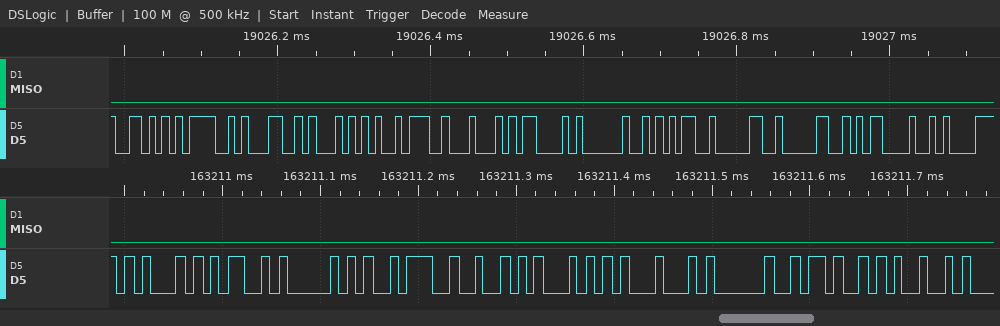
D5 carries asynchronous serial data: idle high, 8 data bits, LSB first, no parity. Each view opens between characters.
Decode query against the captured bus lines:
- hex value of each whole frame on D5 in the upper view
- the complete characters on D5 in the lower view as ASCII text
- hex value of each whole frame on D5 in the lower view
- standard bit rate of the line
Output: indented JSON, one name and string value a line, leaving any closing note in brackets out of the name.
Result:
{
  "hex value of each whole frame on D5 in the upper view": "56, 4F, 4C, 54, 3A, 44, 43, 20, 35, 30, 30, 0D, 0A",
  "the complete characters on D5 in the lower view as ASCII text": "\"EMP:RTD KI\"",
  "hex value of each whole frame on D5 in the lower view": "45, 4D, 50, 3A, 52, 54, 44, 20, 4B, 49",
  "standard bit rate of the line": "115200 baud"
}
